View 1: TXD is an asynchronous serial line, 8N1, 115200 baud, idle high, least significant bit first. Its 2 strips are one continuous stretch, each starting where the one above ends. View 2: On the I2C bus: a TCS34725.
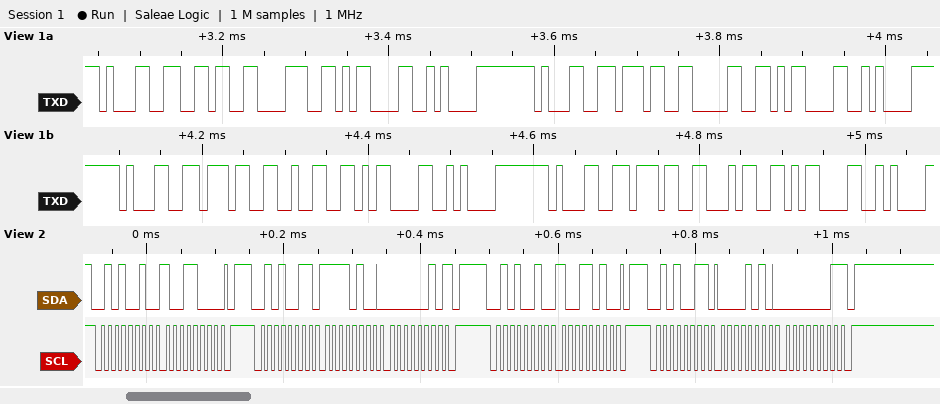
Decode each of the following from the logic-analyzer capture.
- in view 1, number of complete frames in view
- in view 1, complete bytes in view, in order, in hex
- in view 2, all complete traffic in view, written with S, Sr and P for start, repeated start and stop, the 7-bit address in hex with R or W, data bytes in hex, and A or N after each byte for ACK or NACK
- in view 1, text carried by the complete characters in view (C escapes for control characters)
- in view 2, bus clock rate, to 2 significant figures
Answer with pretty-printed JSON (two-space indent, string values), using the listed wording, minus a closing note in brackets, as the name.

{
  "in view 1, number of complete frames in view": "20",
  "in view 1, complete bytes in view, in order, in hex": "31 36 38 0D 0A 31 37 30 0D 0A 31 37 32 0D 0A 31 37 34 0D 0A",
  "in view 2, all complete traffic in view, written with S, Sr and P for start, repeated start and stop, the 7-bit address in hex with R or W, data bytes in hex, and A or N after each byte for ACK or NACK": "S 29W A 98 A P S 29R A F4 A 02 N P S 29W A 9A A P S 29R A 0A A 01 N P",
  "in view 1, text carried by the complete characters in view": "\"168\\r\\n170\\r\\n172\\r\\n174\\r\\n\"",
  "in view 2, bus clock rate, to 2 significant figures": "100 kHz"
}
